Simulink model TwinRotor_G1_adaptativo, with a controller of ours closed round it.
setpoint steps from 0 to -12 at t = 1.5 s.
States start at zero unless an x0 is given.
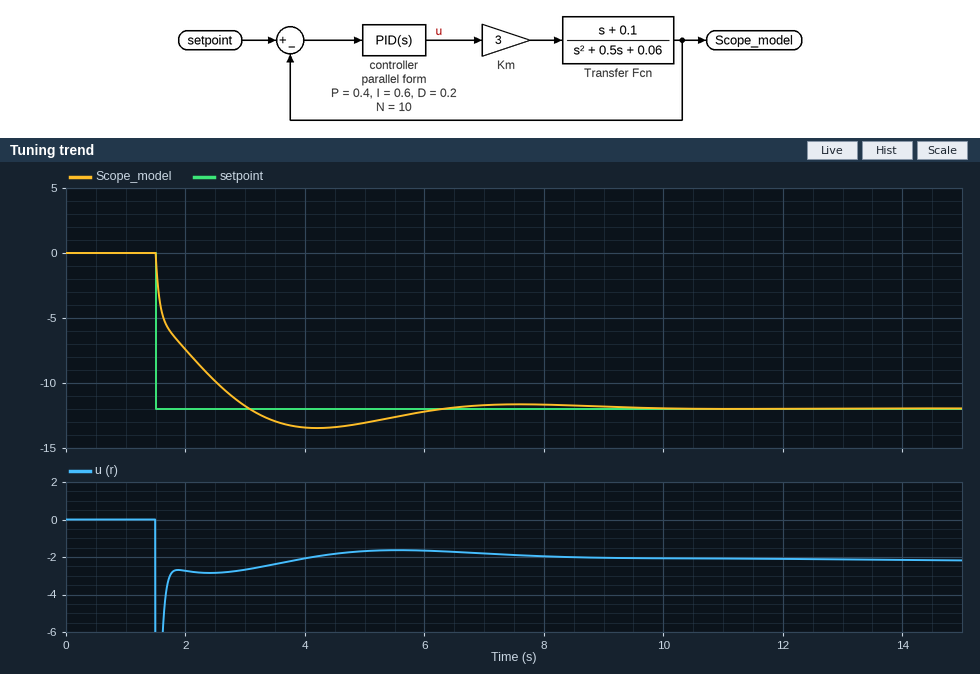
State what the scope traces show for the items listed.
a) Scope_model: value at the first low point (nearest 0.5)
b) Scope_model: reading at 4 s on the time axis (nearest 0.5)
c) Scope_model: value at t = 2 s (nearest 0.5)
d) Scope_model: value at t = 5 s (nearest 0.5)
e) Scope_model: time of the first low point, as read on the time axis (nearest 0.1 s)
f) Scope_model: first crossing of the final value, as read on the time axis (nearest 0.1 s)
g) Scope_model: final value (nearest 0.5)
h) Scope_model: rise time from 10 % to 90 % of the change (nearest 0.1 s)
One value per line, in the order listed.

-13.5
-13.5
-7.5
-13.0
4.2 s
3.1 s
-12.0
1.2 s
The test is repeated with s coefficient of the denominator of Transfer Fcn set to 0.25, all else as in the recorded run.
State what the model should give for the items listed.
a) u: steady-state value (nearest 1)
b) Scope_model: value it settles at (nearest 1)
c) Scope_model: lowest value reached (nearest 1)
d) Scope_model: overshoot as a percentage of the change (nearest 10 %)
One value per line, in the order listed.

-2
-12
-14
20 %
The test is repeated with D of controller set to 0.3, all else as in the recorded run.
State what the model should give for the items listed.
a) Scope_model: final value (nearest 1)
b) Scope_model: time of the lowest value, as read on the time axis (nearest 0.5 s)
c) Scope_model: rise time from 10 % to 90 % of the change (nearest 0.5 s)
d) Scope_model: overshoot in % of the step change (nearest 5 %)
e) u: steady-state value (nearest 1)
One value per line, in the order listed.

-12
4.5 s
1.5 s
10 %
-2
